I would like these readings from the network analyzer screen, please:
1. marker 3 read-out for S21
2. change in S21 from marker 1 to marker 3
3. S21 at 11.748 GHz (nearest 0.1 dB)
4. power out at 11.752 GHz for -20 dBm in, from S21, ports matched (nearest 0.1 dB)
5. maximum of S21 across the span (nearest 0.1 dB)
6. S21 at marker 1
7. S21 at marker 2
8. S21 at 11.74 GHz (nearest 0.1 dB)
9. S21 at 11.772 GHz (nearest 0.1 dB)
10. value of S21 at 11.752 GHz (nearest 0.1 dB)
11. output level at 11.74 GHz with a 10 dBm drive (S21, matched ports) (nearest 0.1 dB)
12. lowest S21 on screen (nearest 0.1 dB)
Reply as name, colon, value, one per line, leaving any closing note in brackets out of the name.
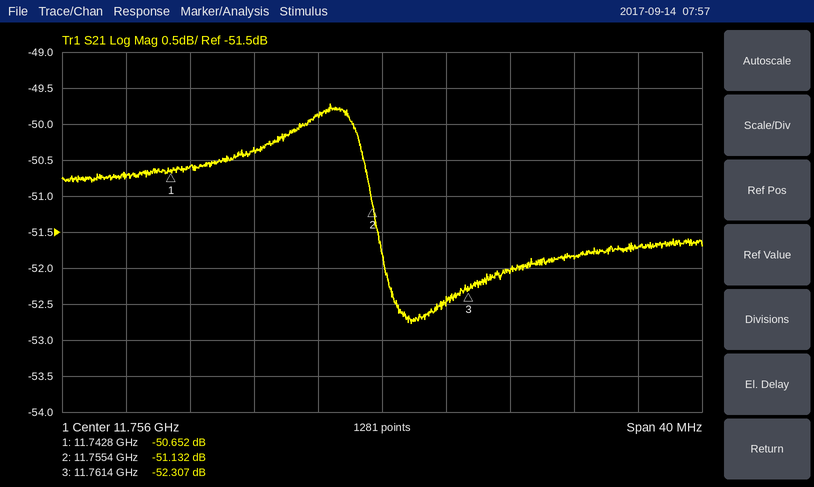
marker 3 read-out for S21: -52.307 dB
change in S21 from marker 1 to marker 3: -1.655 dB
S21 at 11.748 GHz: -50.4 dB
power out at 11.752 GHz for -20 dBm in, from S21, ports matched: -69.9 dBm
maximum of S21 across the span: -49.7 dB
S21 at marker 1: -50.652 dB
S21 at marker 2: -51.132 dB
S21 at 11.74 GHz: -50.7 dB
S21 at 11.772 GHz: -51.7 dB
value of S21 at 11.752 GHz: -49.9 dB
output level at 11.74 GHz with a 10 dBm drive (S21, matched ports): -40.7 dBm
lowest S21 on screen: -52.8 dB
